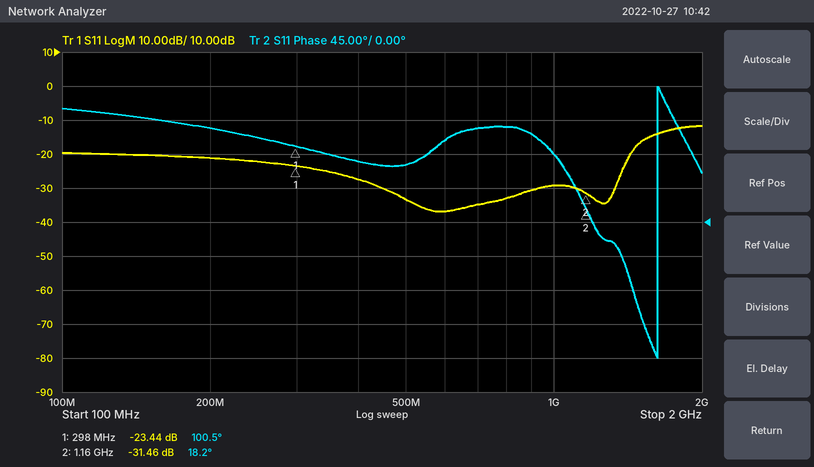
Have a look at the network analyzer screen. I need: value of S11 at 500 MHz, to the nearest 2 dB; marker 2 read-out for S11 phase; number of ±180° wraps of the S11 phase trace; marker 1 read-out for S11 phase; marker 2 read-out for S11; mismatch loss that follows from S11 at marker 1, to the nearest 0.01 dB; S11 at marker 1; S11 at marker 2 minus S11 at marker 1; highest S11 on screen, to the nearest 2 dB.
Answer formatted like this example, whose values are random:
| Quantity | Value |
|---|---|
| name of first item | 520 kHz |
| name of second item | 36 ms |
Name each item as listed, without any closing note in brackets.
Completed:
| Quantity | Value |
|---|---|
| value of S11 at 500 MHz, to the nearest 2 dB | -34 dB |
| marker 2 read-out for S11 phase | 18.2° |
| number of ±180° wraps of the S11 phase trace | 1 |
| marker 1 read-out for S11 phase | 100.5° |
| marker 2 read-out for S11 | -31.46 dB |
| mismatch loss that follows from S11 at marker 1, to the nearest 0.01 dB | 0.02 dB |
| S11 at marker 1 | -23.44 dB |
| S11 at marker 2 minus S11 at marker 1 | -8.02 dB |
| highest S11 on screen, to the nearest 2 dB | -12 dB |
